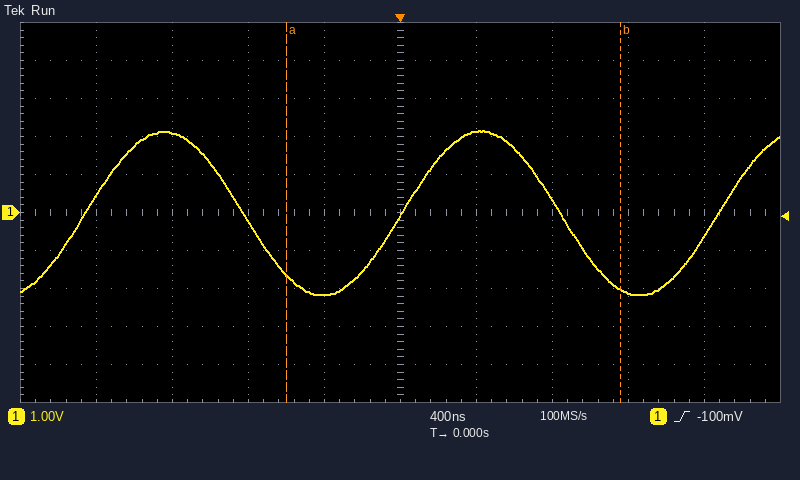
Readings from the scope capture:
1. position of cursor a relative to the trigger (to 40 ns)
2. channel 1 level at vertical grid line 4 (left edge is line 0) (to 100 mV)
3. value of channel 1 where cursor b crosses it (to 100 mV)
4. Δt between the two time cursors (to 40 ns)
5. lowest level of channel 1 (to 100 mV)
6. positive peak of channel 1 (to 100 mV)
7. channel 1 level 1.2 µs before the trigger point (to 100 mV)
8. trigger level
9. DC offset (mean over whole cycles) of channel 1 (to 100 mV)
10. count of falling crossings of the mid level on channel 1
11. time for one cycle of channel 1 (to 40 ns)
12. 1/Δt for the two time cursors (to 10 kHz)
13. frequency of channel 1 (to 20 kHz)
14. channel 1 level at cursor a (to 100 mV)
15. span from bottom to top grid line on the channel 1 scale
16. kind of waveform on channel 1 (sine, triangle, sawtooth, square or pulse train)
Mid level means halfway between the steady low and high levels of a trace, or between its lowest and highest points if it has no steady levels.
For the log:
-600 ns
-2.2 V
-2.0 V
1.76 µs
-2.2 V
2.2 V
2.1 V
-100 mV
0.0 V
2
1.68 µs
570 kHz
600 kHz
-1.6 V
10 V
sine
